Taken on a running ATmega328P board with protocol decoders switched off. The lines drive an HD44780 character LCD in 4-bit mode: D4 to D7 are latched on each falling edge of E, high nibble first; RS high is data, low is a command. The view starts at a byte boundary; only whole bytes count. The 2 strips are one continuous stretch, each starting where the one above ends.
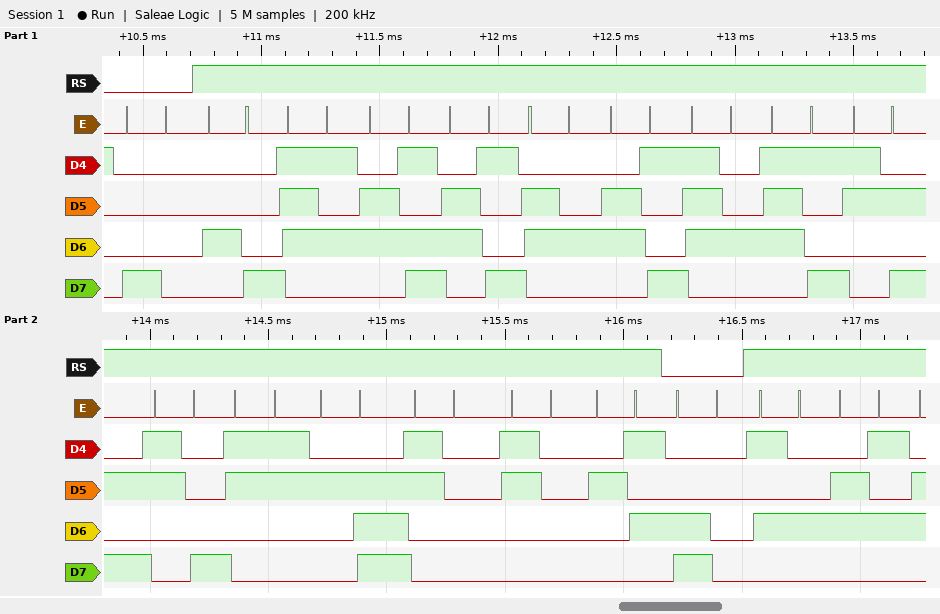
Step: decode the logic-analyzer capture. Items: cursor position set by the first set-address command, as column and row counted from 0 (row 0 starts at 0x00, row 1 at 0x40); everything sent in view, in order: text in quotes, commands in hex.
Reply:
column 0, row 0
0x80 "Humidity:83.00%" 0xC0 "Te"
